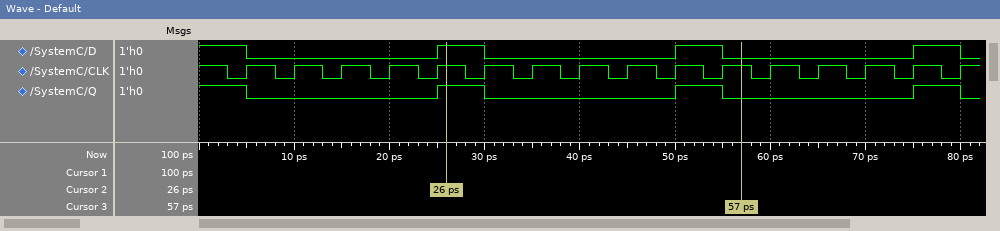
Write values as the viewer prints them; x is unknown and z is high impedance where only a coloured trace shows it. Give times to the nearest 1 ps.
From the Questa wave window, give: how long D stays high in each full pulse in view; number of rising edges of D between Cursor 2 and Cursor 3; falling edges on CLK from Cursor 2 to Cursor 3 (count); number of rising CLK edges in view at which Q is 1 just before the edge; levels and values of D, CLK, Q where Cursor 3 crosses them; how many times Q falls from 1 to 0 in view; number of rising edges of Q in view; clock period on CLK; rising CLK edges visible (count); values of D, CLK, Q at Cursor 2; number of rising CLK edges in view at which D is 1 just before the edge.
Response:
5 ps, 5 ps, 5 ps
1
6
4
D=0, CLK=1, Q=0
4
3
5 ps
16
D=1, CLK=1, Q=1
4
